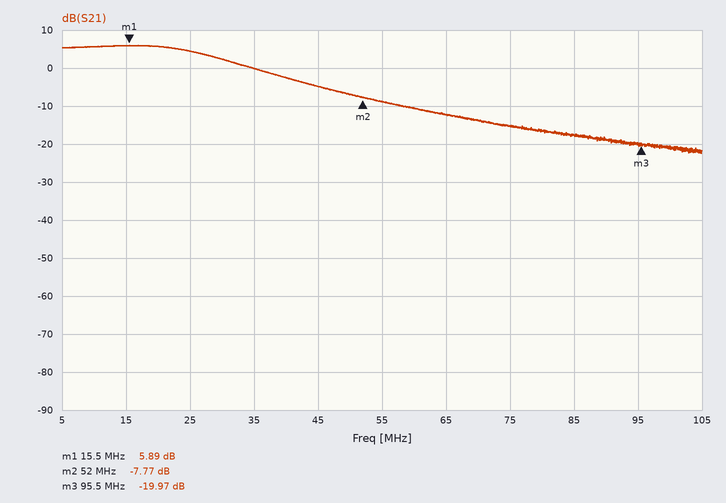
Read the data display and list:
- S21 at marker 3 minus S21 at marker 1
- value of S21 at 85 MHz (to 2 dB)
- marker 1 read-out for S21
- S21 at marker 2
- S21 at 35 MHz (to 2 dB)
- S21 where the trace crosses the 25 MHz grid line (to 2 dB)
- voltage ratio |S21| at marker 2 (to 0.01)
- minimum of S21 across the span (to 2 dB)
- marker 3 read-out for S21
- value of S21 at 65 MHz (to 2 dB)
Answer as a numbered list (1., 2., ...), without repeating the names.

1. -25.86 dB
2. -18 dB
3. 5.89 dB
4. -7.77 dB
5. 0 dB
6. 4 dB
7. 0.41
8. -22 dB
9. -19.97 dB
10. -12 dB
